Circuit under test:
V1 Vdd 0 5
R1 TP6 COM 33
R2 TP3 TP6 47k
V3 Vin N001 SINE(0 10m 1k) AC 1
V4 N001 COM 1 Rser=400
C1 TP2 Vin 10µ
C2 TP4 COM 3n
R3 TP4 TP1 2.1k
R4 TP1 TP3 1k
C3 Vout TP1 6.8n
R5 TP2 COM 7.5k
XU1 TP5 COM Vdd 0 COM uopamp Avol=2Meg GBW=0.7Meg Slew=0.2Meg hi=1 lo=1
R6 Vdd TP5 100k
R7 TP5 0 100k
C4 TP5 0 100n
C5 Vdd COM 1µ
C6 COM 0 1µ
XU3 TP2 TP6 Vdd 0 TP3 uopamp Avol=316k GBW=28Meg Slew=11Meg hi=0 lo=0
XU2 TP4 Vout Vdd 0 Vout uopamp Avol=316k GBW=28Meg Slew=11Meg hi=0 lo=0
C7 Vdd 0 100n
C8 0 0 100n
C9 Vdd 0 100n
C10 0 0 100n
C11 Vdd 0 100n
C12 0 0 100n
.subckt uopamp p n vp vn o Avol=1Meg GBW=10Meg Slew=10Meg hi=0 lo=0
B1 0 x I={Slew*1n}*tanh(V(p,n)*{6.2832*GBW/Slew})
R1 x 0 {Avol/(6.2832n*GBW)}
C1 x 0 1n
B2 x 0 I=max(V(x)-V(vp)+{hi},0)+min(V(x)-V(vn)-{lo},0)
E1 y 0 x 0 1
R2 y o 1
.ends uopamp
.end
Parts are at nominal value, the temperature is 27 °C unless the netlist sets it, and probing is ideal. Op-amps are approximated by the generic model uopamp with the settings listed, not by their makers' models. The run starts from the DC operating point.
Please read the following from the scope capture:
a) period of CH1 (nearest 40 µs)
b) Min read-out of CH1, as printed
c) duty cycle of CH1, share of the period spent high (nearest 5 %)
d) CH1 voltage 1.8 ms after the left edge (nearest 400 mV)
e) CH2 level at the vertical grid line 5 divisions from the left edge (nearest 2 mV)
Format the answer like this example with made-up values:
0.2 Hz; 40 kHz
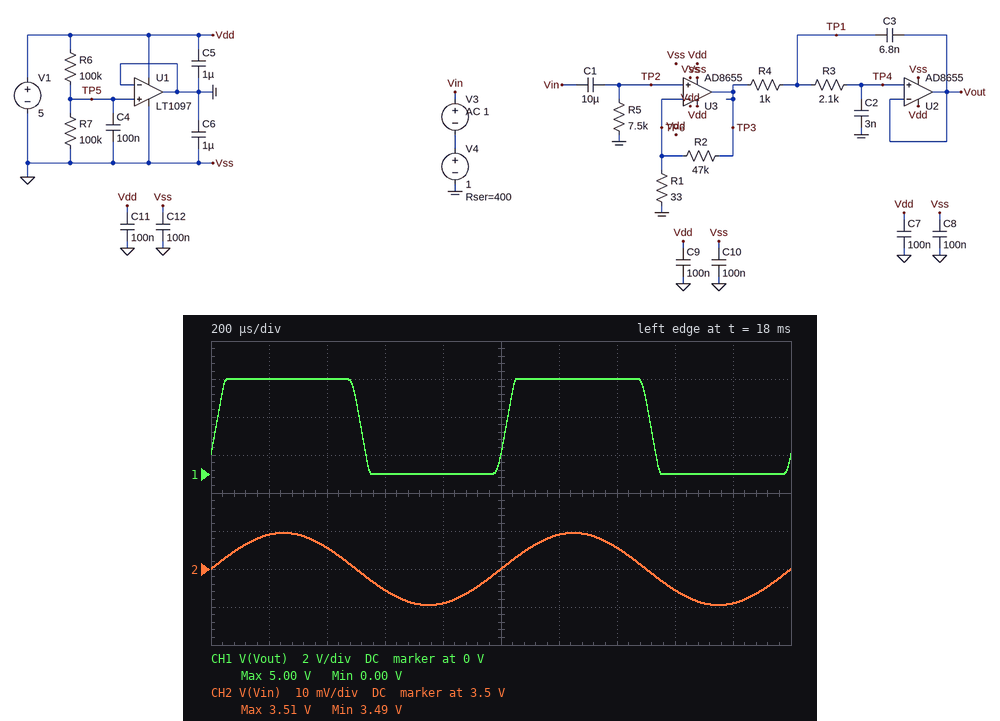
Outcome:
1.00 ms; 0.00 V; 50 %; 0 V; 3.500 V
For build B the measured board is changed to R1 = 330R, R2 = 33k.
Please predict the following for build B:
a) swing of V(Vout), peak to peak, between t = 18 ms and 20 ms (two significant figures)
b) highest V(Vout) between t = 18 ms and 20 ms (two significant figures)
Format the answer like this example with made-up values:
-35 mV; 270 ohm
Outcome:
1.9 V; 3.5 V
